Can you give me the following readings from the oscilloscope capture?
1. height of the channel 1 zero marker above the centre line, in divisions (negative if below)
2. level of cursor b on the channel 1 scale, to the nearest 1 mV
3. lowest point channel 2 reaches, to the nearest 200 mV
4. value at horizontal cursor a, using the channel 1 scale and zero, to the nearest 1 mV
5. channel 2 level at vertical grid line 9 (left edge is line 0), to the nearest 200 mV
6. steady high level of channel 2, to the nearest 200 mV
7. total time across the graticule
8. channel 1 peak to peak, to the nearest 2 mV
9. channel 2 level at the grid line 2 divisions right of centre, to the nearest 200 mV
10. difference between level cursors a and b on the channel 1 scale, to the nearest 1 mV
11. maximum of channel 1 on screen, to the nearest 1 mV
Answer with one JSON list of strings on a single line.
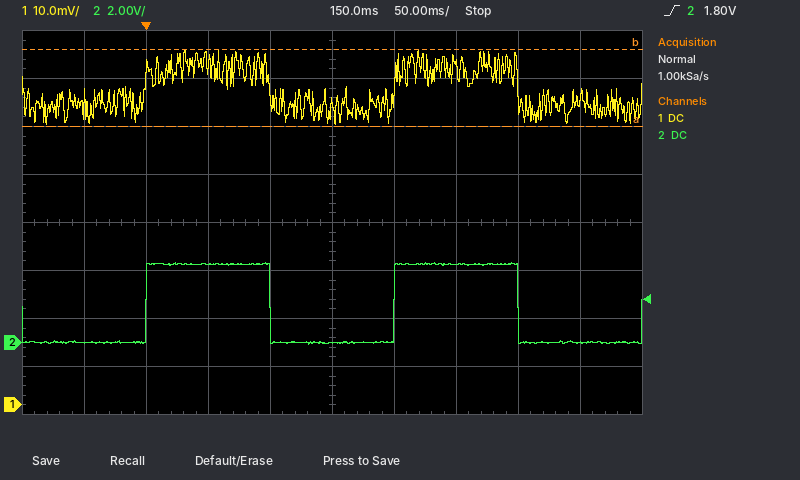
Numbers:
["-3.8 div", "74 mV", "0.0 V", "58 mV", "0.0 V", "3.2 V", "500 ms", "16 mV", "3.2 V", "16 mV", "74 mV"]
